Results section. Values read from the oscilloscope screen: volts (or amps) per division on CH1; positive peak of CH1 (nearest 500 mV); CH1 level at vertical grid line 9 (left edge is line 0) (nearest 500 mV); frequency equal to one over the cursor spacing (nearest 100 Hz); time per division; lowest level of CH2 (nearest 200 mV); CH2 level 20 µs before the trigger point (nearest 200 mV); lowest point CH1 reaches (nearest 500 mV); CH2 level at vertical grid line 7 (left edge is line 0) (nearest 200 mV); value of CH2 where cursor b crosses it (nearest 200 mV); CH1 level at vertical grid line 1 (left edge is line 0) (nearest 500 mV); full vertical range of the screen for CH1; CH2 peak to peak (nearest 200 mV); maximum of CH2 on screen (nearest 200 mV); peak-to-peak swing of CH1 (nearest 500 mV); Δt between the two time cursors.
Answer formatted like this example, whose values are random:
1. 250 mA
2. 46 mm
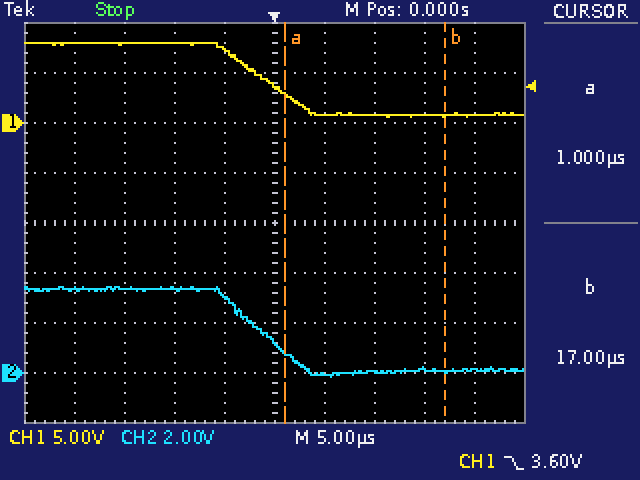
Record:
1. 5 V
2. 8.0 V
3. 1.0 V
4. 62.5 kHz
5. 5 µs
6. -200 mV
7. 3.4 V
8. 500 mV
9. 0.0 V
10. 0.0 V
11. 8.0 V
12. 40 V
13. 3.6 V
14. 3.4 V
15. 7.5 V
16. 16.0 µs
